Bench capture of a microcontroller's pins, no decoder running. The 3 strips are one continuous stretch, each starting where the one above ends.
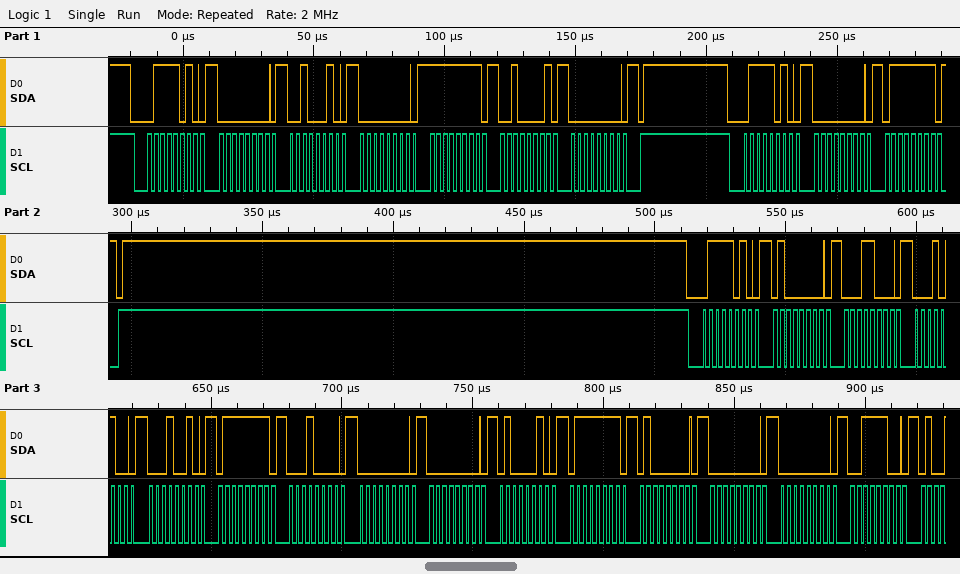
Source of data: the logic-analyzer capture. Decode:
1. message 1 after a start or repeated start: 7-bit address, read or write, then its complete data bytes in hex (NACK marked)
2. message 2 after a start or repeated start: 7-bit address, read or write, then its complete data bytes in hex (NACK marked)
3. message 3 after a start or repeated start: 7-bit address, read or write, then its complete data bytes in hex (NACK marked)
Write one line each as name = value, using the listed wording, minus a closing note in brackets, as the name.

message 1 after a start or repeated start: 7-bit address, read or write, then its complete data bytes in hex = 0x3D write: 00 22 00 FF 21 00
message 2 after a start or repeated start: 7-bit address, read or write, then its complete data bytes in hex = 0x3D write: 00 7F
message 3 after a start or repeated start: 7-bit address, read or write, then its complete data bytes in hex = 0x3D write: 40 18 14 12 7F 10 00 00 42 7F 40 00 00 3C
